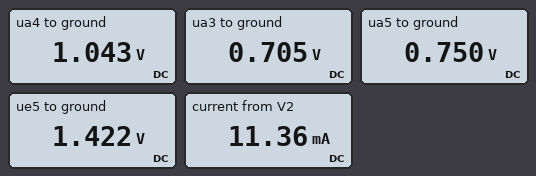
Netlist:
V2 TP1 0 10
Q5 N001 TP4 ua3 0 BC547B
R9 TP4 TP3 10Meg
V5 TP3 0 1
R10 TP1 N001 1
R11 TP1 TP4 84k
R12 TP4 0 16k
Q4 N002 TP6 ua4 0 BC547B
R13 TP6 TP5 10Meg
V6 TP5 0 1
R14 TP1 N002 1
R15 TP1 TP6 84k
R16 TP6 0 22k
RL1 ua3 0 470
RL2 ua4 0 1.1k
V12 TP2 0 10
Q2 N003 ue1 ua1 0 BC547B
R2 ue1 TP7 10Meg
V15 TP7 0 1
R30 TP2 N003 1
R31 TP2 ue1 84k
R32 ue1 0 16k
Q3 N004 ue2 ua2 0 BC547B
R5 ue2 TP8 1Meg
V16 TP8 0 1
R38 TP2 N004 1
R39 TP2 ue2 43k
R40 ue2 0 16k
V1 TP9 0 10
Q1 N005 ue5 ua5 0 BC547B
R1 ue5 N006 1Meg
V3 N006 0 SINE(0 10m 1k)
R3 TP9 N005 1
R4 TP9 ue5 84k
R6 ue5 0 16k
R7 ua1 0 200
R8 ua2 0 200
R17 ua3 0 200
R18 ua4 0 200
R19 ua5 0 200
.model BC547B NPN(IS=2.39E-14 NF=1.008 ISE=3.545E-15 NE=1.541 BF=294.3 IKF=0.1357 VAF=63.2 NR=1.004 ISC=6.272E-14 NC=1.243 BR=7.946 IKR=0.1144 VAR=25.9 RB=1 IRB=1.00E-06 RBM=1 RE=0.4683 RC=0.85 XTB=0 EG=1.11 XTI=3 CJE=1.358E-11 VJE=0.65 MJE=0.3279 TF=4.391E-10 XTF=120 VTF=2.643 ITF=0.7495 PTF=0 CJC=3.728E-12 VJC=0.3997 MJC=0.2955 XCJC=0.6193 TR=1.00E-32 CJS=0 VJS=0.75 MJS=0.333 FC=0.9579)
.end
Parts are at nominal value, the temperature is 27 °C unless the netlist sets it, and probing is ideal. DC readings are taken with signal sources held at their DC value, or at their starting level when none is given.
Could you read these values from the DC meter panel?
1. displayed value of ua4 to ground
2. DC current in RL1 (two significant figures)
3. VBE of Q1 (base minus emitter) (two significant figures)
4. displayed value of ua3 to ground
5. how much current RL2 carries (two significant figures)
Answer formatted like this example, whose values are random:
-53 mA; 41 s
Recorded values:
1.043 V; 1.5 mA; 670 mV; 0.705 V; 950 µA
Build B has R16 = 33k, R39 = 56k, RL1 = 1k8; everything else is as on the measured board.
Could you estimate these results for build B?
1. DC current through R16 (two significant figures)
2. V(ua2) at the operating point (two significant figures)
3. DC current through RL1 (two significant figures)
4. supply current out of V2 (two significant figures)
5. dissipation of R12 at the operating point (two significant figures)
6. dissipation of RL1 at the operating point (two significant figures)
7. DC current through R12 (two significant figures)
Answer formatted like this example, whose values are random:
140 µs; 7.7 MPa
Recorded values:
65 µA; 1.3 V; 420 µA; 13 mA; 130 µW; 310 µW; 89 µA
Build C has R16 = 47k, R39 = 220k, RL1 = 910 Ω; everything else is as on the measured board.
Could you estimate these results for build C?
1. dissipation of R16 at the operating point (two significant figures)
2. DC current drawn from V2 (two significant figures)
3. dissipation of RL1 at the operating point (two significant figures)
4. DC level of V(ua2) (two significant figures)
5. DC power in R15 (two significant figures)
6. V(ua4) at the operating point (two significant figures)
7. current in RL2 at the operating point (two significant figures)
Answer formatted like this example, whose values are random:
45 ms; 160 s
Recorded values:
130 µW; 15 mA; 590 µW; 64 mV; 670 µW; 1.8 V; 1.6 mA
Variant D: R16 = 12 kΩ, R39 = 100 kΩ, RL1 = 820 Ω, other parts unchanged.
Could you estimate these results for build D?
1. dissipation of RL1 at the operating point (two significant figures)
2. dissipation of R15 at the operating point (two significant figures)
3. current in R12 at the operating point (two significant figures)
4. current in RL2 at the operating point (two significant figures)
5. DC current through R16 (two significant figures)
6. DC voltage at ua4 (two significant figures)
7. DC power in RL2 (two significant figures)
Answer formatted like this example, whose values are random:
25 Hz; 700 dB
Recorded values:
650 µW; 930 µW; 88 µA; 450 µA; 96 µA; 490 mV; 220 µW
